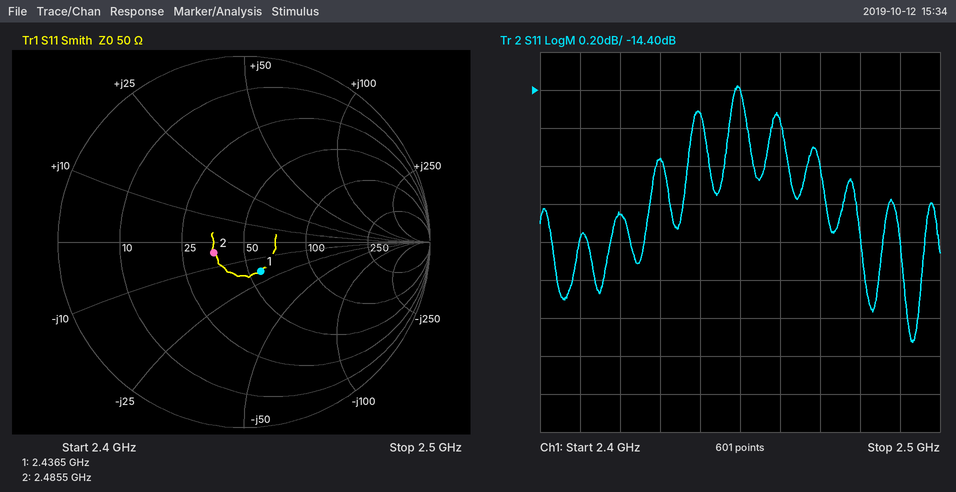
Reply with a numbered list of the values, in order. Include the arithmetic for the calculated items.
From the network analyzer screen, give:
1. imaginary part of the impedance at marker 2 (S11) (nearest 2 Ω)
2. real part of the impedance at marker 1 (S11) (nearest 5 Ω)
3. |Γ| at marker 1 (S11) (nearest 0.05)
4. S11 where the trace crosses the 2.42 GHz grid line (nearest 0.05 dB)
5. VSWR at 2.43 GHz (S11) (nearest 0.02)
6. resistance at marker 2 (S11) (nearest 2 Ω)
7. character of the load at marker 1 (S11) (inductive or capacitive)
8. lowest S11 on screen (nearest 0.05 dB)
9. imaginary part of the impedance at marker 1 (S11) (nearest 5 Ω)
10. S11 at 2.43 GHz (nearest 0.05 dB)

1. -4 Ω
2. 55 Ω
3. 0.20
4. -15.05 dB
5. |Γ| = 10^(-14.75/20) = 0.1830; VSWR = (1 + 0.1830)/(1 − 0.1830) ≈ 1.45, so 1.44 to the nearest 0.02
6. 36 Ω
7. capacitive
8. -15.75 dB
9. -20 Ω
10. -14.75 dB
